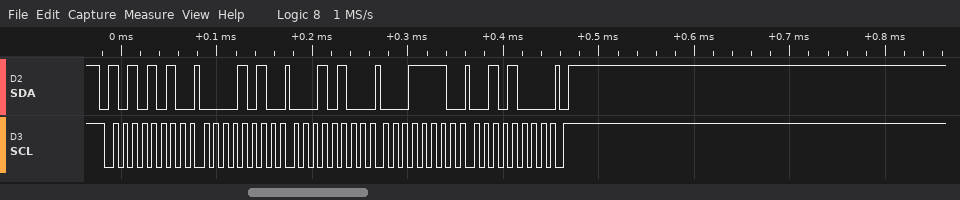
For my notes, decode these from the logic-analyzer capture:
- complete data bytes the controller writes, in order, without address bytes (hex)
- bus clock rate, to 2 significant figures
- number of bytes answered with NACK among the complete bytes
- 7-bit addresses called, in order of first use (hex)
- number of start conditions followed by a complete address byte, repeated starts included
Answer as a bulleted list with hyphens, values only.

- 0A 14 1E 28
- 100 kHz
- 0
- 0x55
- 1
